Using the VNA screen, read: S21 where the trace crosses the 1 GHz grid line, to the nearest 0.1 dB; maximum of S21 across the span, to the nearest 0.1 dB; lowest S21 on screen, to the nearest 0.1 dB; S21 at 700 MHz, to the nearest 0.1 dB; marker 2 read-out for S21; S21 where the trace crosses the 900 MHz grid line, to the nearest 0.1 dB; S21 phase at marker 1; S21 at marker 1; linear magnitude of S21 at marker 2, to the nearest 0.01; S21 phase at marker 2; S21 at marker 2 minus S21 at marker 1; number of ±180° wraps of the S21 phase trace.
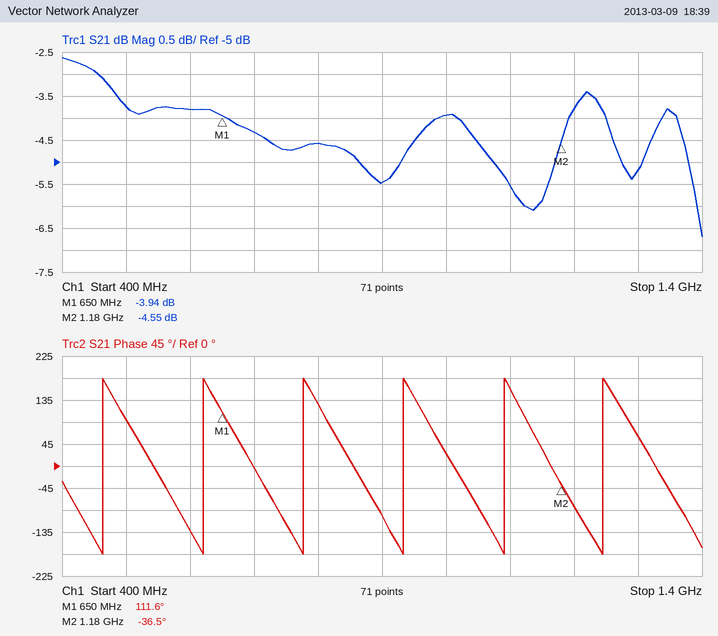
-3.9 dB
-2.6 dB
-6.7 dB
-4.3 dB
-4.55 dB
-5.5 dB
111.6°
-3.94 dB
0.59
-36.5°
-0.61 dB
6
